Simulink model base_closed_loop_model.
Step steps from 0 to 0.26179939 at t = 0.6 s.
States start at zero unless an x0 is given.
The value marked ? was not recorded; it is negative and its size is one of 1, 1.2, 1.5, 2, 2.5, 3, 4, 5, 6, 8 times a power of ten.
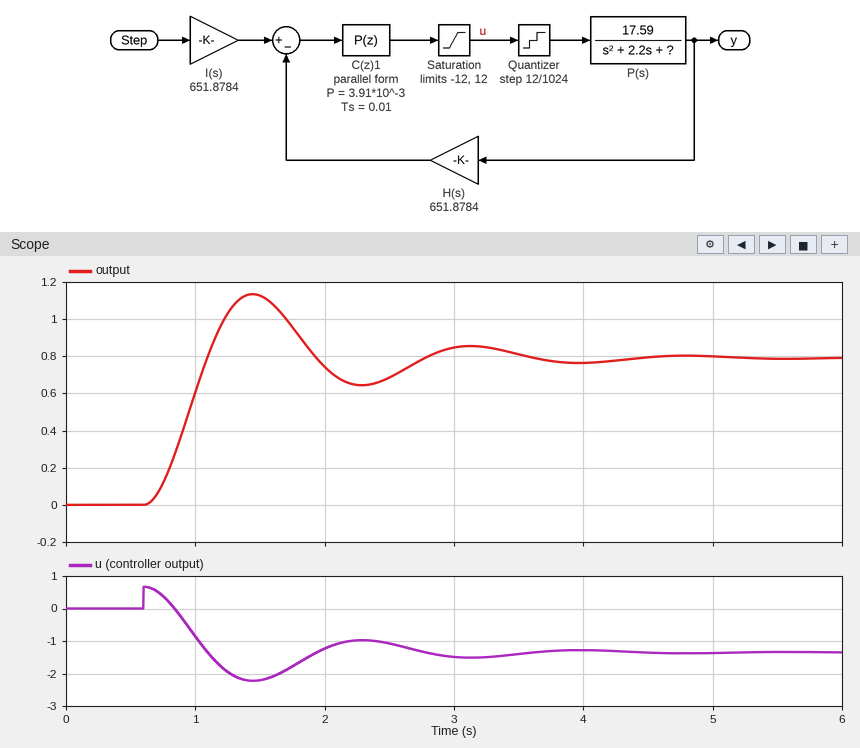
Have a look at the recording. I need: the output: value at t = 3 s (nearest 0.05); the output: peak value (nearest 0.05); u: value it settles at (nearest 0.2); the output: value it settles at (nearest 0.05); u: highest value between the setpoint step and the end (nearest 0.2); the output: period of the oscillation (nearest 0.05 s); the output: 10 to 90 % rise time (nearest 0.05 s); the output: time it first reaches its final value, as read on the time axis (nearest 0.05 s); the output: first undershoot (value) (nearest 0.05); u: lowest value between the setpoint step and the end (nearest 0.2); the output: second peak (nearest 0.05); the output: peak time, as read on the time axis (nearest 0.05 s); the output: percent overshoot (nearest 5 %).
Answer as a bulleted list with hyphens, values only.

- 0.85
- 1.15
- -1.4
- 0.80
- 0.6
- 1.70 s
- 0.35 s
- 1.10 s
- 0.65
- -2.2
- 0.85
- 1.45 s
- 45 %
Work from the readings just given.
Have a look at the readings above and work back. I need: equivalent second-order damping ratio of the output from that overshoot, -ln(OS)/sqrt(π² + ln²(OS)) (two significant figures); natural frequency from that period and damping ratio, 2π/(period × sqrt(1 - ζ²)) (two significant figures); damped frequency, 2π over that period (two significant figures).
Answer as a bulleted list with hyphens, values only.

- 0.25
- 3.8 rad/s
- 3.7 rad/s
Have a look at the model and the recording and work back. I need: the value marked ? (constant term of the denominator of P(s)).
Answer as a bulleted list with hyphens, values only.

- -30
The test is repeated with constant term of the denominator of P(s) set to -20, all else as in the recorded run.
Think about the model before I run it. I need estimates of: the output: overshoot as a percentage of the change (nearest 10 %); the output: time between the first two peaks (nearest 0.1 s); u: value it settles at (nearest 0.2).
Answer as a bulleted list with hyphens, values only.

- 50 %
- 1.3 s
- -0.6
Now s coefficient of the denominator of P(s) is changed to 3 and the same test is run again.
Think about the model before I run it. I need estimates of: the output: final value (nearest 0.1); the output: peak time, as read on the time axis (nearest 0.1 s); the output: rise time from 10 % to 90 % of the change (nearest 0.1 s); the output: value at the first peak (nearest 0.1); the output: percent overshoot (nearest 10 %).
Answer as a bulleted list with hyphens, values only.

- 0.8
- 1.5 s
- 0.4 s
- 1.0
- 30 %
